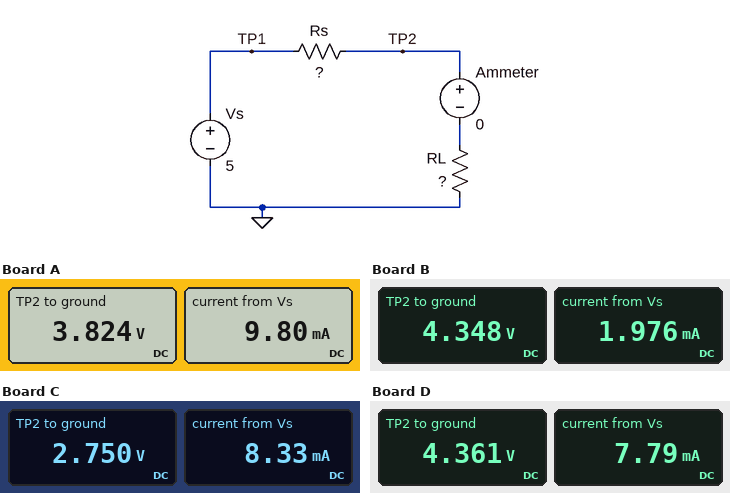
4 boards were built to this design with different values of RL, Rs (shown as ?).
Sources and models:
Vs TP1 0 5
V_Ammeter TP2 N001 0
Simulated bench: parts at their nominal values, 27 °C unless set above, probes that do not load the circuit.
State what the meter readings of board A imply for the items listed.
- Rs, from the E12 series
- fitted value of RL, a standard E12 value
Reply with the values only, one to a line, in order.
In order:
120 Ω
390 Ω
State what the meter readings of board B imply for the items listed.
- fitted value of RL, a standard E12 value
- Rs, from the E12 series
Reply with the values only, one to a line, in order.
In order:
2.2 kΩ
330 Ω
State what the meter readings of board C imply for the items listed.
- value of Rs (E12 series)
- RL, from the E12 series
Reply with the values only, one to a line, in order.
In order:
270 Ω
330 Ω
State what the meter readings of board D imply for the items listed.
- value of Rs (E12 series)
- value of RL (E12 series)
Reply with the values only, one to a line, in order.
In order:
82 Ω
560 Ω
